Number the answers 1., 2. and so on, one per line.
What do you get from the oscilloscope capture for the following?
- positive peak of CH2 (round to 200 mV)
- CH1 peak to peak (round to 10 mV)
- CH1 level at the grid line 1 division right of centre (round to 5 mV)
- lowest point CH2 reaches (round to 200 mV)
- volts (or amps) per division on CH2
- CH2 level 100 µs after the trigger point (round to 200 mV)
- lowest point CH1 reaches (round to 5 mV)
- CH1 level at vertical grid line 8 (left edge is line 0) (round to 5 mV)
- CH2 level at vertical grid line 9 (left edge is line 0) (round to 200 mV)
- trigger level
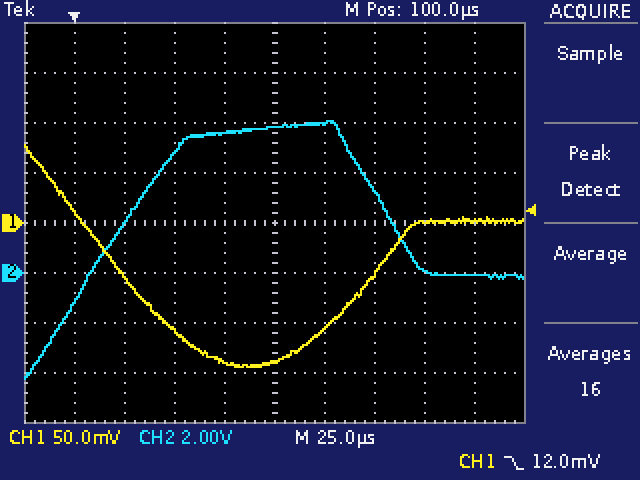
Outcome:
1. 6.0 V
2. 220 mV
3. -105 mV
4. -4.2 V
5. 2 V
6. 5.8 V
7. -145 mV
8. 0 mV
9. 0.0 V
10. 12.0 mV
